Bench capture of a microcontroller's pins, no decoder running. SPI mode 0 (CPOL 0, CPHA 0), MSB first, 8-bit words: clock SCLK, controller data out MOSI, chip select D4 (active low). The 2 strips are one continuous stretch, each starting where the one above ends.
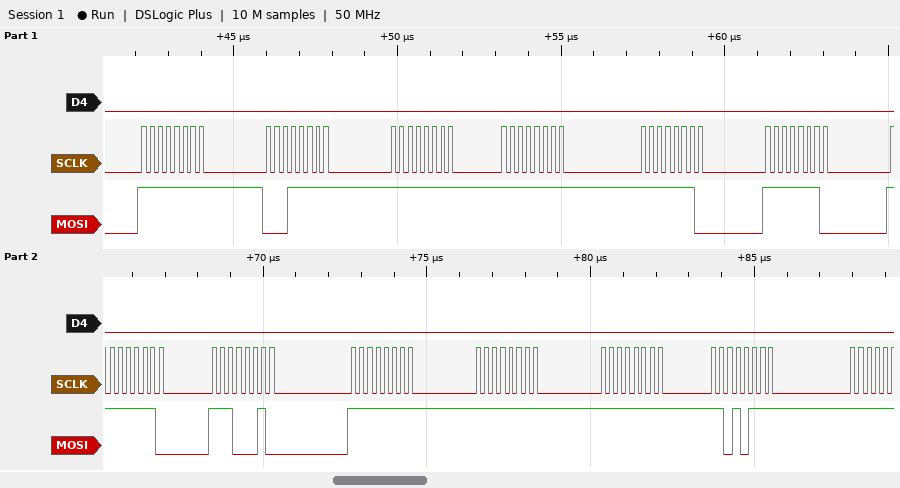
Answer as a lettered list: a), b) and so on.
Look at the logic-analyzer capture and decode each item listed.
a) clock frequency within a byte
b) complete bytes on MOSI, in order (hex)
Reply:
a) 4 MHz
b) FF 1F FF FF FE FE FE E2 FF FF FF D7
